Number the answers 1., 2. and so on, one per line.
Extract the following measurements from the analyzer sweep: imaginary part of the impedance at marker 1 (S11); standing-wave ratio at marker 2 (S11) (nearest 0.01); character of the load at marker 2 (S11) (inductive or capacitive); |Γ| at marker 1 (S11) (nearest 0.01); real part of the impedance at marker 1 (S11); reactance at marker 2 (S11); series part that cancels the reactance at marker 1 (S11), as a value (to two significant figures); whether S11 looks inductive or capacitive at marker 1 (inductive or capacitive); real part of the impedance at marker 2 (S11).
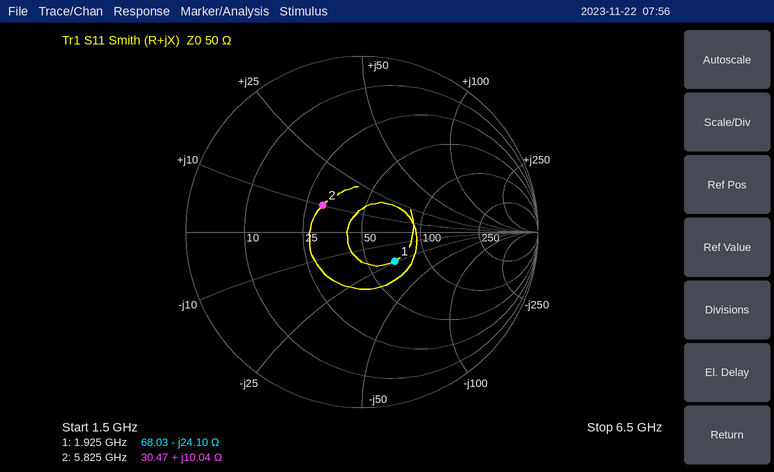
1. -24.10 Ω
2. 1.74
3. inductive
4. 0.25
5. 68.03 Ω
6. +10.04 Ω
7. 2.0 nH
8. capacitive
9. 30.47 Ω
